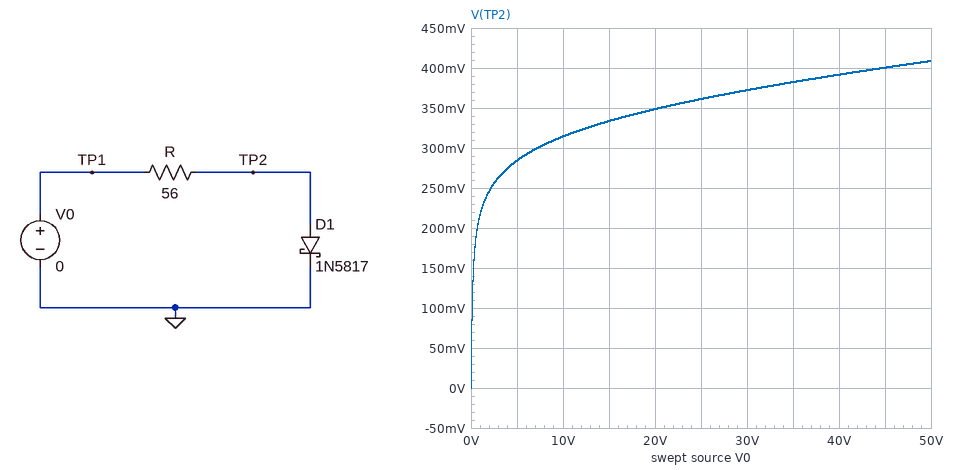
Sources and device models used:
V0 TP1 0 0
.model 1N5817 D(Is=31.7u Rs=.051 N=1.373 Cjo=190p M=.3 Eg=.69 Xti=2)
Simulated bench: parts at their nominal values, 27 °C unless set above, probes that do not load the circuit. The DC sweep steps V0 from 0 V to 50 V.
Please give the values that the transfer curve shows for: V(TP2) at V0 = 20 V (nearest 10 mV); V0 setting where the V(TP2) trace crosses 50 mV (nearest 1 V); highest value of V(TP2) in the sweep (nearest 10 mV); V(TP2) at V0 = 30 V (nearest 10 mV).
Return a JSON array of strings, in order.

["350 mV", "0 V", "410 mV", "370 mV"]
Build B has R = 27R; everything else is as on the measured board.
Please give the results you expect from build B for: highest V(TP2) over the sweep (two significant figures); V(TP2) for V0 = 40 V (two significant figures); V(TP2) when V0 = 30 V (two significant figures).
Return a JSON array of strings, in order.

["480 mV", "460 mV", "430 mV"]
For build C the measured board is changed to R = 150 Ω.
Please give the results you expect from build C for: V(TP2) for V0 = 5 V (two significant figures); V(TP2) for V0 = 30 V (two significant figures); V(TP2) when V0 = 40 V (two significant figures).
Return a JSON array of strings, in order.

["250 mV", "320 mV", "330 mV"]
